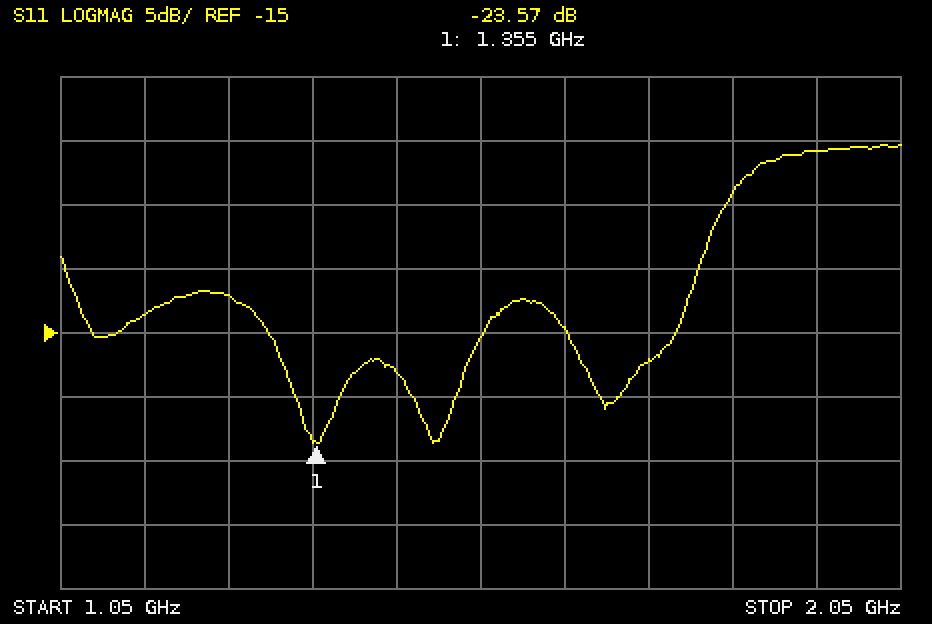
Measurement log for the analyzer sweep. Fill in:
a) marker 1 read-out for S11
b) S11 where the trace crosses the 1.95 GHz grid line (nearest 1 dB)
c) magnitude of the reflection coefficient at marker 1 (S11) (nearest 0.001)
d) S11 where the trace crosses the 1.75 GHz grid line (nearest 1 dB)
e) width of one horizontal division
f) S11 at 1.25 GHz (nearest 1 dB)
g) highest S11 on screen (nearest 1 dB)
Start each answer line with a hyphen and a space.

- -23.57 dB
- -1 dB
- 0.066
- -17 dB
- 100 MHz
- -12 dB
- 0 dB
